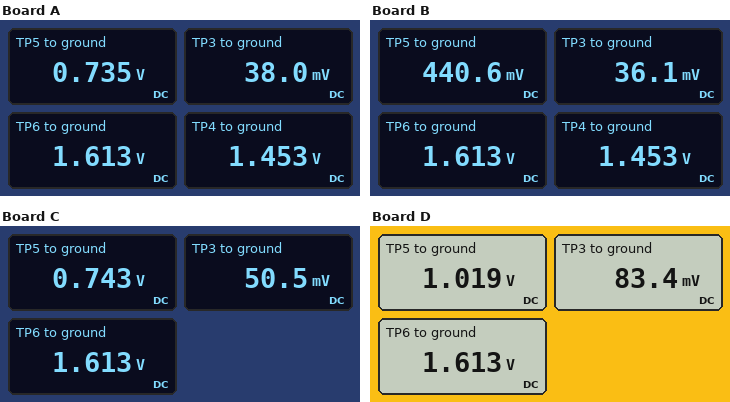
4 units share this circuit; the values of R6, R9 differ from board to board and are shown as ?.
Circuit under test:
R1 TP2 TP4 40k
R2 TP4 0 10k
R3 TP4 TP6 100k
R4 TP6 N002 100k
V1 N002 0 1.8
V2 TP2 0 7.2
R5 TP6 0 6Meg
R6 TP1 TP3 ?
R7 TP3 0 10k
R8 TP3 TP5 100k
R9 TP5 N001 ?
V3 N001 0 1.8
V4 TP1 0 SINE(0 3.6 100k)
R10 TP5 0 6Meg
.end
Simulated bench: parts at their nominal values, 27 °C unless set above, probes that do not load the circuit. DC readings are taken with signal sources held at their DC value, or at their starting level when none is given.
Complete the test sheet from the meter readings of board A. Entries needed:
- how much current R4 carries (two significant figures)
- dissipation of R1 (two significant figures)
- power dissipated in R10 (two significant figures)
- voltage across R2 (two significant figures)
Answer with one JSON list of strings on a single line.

["1.9 µA", "830 µW", "90 nW", "1.5 V"]
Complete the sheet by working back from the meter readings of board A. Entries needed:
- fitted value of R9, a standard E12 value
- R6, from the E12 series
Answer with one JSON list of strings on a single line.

["150 kΩ", "12 kΩ"]
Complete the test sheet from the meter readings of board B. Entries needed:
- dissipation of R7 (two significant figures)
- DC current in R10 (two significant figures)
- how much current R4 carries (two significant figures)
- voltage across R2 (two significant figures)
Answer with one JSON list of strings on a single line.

["130 nW", "73 nA", "1.9 µA", "1.5 V"]
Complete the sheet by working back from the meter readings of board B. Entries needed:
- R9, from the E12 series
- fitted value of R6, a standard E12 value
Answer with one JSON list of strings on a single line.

["330 kΩ", "82 kΩ"]
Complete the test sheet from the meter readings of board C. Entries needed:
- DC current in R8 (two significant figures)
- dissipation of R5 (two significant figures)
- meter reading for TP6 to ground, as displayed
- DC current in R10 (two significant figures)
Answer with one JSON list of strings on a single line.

["6.9 µA", "430 nW", "1.613 V", "120 nA"]
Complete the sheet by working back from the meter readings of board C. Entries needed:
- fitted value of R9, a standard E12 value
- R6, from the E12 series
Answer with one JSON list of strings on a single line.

["150 kΩ", "27 kΩ"]
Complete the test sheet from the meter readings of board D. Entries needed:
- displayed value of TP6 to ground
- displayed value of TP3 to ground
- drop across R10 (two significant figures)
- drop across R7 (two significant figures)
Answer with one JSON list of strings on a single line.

["1.613 V", "83.4 mV", "1.0 V", "83 mV"]
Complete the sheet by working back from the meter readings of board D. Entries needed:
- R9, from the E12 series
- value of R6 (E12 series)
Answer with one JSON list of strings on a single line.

["82 kΩ", "82 kΩ"]
